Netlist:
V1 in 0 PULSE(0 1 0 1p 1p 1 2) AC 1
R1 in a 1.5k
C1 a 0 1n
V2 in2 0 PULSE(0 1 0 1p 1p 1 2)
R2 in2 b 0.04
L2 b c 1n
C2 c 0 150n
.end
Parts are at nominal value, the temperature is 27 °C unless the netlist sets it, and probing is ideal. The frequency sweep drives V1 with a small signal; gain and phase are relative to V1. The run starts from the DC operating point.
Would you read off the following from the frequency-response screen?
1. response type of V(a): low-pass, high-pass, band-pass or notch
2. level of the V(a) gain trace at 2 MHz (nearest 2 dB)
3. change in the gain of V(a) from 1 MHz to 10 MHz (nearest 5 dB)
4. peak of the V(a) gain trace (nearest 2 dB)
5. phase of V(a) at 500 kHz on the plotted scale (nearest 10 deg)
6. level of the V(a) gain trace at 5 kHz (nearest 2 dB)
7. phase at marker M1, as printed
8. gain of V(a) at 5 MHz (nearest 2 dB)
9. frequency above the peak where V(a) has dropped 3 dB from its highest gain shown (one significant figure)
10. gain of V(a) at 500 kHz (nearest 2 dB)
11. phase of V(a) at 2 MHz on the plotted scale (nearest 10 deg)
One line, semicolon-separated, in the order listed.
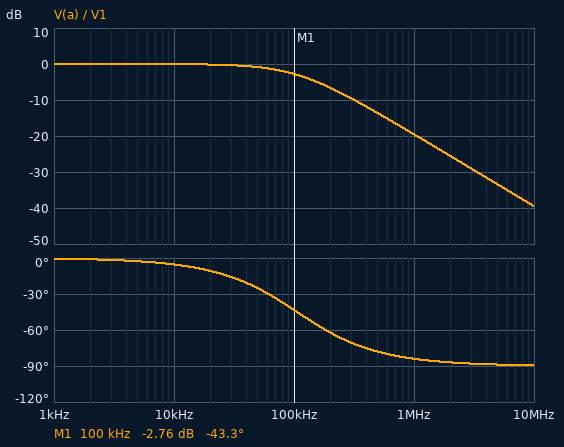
low-pass; -26 dB; -20 dB; 0 dB; -80 deg; 0 dB; -43.3 deg; -34 dB; 100 kHz; -14 dB; -90 deg
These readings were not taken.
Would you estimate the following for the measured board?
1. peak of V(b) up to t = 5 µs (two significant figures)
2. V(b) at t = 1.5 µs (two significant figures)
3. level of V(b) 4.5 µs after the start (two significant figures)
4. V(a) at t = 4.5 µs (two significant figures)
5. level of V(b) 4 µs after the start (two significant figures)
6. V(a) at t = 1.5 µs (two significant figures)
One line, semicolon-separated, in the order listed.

1.2 V; 1.0 V; 1.0 V; 950 mV; 1.0 V; 630 mV
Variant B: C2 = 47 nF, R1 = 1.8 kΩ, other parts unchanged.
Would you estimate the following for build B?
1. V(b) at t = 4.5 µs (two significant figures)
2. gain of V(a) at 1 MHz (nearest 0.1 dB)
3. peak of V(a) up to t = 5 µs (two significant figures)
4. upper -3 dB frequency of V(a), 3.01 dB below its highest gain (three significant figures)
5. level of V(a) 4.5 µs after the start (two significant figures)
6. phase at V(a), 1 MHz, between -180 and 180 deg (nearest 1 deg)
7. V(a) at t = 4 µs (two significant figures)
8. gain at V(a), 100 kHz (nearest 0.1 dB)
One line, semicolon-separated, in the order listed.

1.0 V; -21.1 dB; 940 mV; 88.4 kHz; 920 mV; -85 deg; 890 mV; -3.6 dB
